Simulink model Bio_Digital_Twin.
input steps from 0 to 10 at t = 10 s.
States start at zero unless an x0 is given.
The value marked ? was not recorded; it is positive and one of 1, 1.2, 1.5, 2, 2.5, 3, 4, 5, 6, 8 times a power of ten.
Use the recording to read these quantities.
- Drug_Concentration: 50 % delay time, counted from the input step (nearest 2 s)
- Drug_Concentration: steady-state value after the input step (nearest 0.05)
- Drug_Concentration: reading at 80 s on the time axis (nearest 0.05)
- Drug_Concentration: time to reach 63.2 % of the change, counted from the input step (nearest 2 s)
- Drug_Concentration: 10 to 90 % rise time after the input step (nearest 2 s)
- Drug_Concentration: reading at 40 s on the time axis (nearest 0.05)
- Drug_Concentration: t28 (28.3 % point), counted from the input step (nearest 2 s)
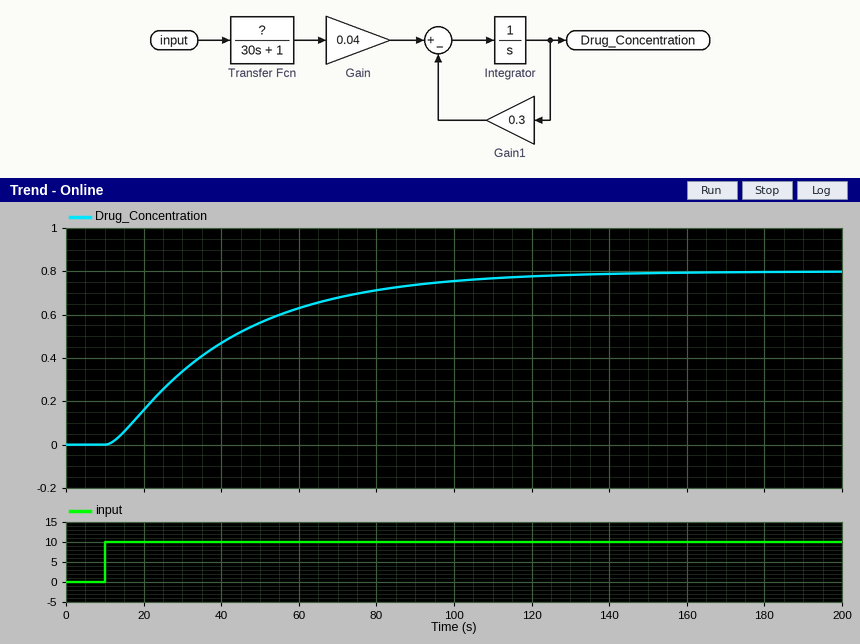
24 s
0.80
0.70
34 s
66 s
0.45
14 s
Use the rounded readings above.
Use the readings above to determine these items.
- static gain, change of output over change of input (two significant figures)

0.080
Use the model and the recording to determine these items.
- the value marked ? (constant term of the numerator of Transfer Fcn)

0.6
